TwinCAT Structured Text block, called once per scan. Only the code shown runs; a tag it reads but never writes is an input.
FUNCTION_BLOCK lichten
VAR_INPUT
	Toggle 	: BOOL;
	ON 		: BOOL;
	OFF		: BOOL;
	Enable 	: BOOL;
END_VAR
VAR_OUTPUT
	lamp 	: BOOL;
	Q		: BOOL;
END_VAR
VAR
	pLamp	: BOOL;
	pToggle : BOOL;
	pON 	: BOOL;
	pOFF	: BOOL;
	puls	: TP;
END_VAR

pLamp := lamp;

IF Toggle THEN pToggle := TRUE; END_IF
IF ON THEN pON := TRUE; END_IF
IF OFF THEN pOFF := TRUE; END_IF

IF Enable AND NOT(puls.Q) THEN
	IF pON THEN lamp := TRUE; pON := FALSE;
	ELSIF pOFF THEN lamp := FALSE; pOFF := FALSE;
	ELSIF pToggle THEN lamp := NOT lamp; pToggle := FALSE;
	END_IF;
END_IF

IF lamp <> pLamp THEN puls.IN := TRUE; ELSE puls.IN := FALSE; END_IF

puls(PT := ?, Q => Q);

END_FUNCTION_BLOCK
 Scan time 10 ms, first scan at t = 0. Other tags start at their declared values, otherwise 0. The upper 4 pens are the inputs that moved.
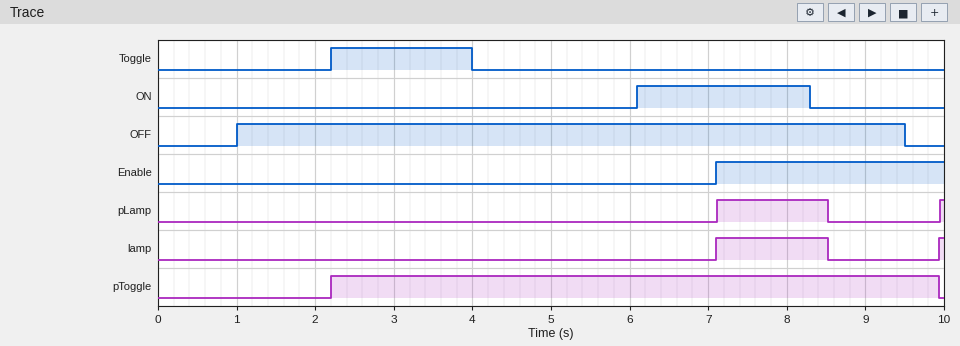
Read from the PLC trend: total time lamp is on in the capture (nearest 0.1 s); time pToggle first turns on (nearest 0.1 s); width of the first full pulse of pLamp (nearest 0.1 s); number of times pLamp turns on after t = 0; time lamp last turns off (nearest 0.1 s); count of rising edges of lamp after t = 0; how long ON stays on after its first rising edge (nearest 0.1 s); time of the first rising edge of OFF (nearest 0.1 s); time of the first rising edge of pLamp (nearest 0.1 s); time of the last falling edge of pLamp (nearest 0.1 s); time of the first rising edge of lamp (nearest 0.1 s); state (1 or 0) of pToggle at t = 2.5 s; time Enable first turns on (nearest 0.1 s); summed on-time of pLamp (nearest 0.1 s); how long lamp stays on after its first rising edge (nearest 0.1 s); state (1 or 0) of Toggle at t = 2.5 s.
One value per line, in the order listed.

1.5 s
2.2 s
1.4 s
2
8.5 s
2
2.2 s
1.0 s
7.1 s
8.5 s
7.1 s
1
7.1 s
1.5 s
1.4 s
1
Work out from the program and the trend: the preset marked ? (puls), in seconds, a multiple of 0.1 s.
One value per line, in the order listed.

1.4 s
